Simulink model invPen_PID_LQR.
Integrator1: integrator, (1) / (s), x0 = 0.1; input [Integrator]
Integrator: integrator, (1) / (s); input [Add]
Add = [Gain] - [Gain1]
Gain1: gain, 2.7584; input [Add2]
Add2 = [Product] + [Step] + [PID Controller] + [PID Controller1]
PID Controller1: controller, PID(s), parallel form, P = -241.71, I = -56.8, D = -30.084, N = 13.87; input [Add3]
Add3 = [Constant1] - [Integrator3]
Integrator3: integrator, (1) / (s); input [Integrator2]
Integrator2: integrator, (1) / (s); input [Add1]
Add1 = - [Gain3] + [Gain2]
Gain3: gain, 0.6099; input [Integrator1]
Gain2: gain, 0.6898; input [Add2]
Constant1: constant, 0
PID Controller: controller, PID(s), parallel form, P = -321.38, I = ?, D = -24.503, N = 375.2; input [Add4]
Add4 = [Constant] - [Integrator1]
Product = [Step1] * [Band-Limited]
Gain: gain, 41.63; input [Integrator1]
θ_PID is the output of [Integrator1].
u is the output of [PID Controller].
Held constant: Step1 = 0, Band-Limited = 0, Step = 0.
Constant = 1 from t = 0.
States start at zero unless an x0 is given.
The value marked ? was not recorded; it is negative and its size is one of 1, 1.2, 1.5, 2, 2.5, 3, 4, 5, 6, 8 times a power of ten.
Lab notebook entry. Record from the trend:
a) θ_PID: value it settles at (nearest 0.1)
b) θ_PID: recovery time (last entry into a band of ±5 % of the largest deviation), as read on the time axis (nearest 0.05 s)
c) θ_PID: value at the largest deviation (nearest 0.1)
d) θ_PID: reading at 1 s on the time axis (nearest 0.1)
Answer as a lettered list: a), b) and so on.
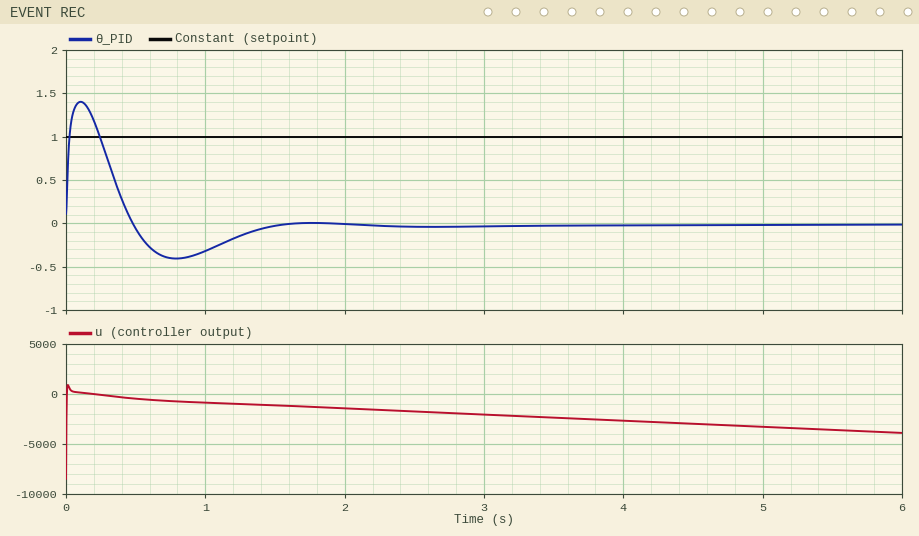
a) 0.0
b) 1.40 s
c) 1.4
d) -0.3
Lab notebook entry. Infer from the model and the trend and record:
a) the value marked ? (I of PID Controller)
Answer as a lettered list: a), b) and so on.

a) -600
